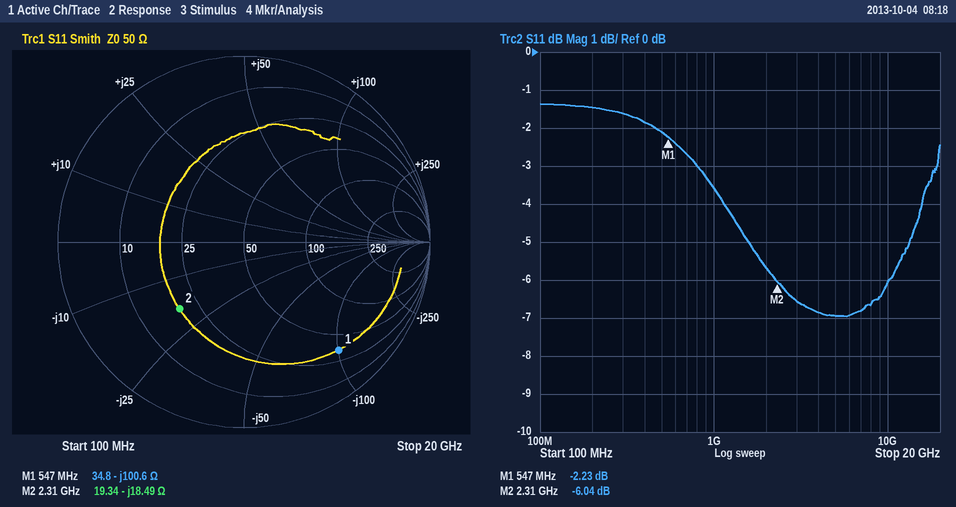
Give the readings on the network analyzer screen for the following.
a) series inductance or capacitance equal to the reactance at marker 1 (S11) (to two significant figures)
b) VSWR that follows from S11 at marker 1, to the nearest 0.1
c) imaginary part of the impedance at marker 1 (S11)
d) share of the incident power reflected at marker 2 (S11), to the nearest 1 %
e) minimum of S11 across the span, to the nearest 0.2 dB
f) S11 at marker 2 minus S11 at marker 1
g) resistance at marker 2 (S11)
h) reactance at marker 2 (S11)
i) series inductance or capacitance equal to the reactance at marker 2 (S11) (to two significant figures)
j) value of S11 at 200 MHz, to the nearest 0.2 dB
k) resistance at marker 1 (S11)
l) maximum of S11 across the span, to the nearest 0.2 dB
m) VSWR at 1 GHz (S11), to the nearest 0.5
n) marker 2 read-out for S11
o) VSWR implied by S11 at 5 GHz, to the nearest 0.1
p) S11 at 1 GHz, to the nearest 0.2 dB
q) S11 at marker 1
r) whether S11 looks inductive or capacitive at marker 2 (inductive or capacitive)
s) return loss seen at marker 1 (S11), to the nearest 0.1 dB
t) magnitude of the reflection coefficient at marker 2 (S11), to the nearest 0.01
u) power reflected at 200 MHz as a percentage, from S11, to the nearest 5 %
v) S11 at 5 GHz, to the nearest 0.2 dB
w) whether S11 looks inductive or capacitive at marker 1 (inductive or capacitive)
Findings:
2.9 pF
7.8
-100.6 Ω
25 %
-7.0 dB
-3.81 dB
19.34 Ω
-18.49 Ω
3.7 pF
-1.4 dB
34.8 Ω
-1.4 dB
5.0
-6.04 dB
2.6
-3.6 dB
-2.23 dB
capacitive
2.2 dB
0.50
70 %
-7.0 dB
capacitive
